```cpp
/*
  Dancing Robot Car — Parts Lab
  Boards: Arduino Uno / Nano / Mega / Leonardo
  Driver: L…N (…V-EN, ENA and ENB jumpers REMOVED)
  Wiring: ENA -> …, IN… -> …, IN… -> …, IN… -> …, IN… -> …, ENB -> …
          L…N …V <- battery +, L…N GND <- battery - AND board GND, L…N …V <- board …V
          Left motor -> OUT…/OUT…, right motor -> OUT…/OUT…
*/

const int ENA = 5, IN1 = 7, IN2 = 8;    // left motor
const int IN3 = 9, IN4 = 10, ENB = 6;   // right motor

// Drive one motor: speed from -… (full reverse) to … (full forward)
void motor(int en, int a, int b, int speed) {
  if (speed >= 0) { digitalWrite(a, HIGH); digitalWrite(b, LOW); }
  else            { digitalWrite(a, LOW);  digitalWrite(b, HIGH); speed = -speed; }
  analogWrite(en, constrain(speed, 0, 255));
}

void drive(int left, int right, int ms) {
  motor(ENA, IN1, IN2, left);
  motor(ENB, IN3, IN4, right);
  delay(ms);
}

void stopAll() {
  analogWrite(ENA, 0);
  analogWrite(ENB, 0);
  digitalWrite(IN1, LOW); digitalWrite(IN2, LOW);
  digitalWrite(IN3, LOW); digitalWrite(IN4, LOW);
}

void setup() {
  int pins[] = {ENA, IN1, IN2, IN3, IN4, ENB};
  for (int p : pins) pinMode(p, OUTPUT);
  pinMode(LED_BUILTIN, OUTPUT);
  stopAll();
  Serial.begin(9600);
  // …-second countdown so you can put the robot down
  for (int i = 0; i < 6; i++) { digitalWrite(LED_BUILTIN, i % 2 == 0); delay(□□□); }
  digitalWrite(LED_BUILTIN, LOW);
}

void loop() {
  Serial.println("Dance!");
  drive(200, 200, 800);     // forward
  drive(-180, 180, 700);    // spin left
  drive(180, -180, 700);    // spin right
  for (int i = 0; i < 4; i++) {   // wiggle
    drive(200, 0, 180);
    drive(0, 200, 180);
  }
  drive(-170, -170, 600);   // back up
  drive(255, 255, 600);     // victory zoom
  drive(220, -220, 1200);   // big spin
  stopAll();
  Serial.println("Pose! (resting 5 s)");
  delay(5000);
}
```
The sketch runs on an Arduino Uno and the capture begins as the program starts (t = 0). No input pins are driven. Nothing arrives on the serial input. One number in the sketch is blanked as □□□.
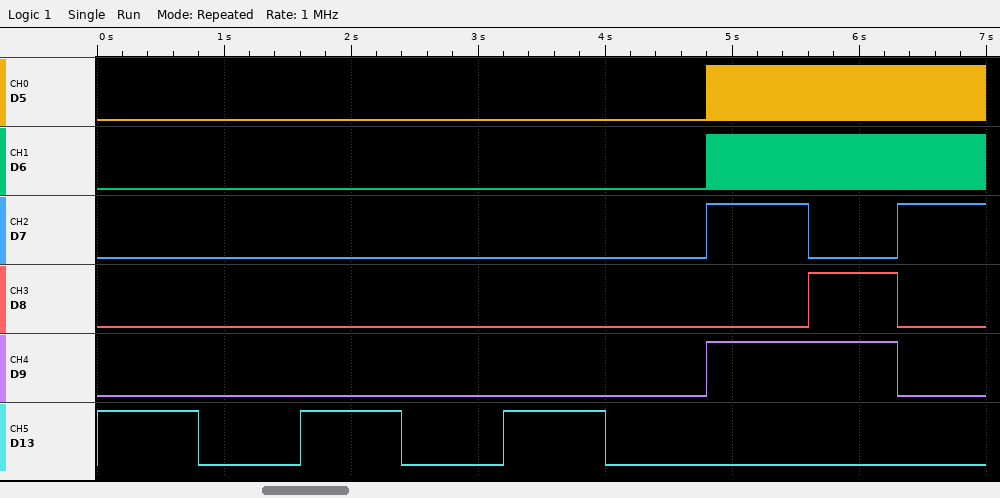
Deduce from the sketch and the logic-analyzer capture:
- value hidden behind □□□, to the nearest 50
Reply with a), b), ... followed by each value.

a) 800
